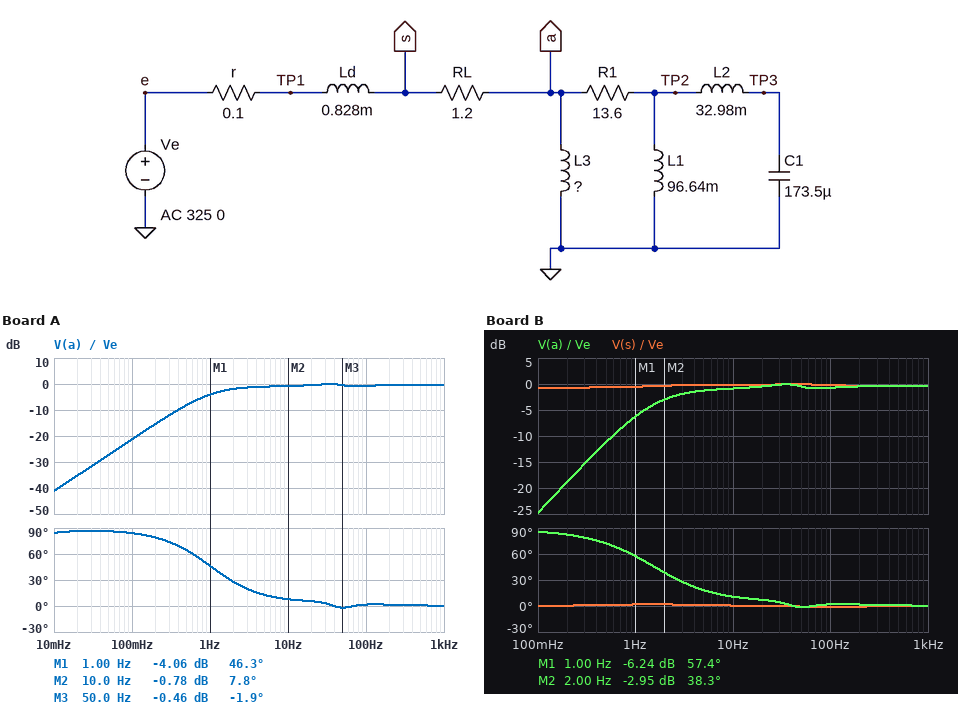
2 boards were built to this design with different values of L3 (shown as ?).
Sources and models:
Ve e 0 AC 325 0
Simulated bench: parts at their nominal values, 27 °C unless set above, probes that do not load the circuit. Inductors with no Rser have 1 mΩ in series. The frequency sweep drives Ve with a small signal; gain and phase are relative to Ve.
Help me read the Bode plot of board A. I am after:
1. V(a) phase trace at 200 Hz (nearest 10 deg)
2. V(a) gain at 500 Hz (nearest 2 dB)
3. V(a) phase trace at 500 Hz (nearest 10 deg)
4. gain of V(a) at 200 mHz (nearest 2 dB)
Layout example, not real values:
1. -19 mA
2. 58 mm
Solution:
1. 0 deg
2. 0 dB
3. 0 deg
4. -16 dB
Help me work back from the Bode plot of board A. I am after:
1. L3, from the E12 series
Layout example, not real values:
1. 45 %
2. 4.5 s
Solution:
1. 180 mH
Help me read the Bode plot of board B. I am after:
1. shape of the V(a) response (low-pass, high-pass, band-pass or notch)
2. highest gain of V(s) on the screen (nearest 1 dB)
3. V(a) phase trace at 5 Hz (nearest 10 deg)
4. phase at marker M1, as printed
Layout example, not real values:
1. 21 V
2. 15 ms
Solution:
1. high-pass
2. 0 dB
3. 20 deg
4. 57.4 deg
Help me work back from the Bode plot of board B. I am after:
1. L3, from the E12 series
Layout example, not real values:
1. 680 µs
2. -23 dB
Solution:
1. 120 mH
